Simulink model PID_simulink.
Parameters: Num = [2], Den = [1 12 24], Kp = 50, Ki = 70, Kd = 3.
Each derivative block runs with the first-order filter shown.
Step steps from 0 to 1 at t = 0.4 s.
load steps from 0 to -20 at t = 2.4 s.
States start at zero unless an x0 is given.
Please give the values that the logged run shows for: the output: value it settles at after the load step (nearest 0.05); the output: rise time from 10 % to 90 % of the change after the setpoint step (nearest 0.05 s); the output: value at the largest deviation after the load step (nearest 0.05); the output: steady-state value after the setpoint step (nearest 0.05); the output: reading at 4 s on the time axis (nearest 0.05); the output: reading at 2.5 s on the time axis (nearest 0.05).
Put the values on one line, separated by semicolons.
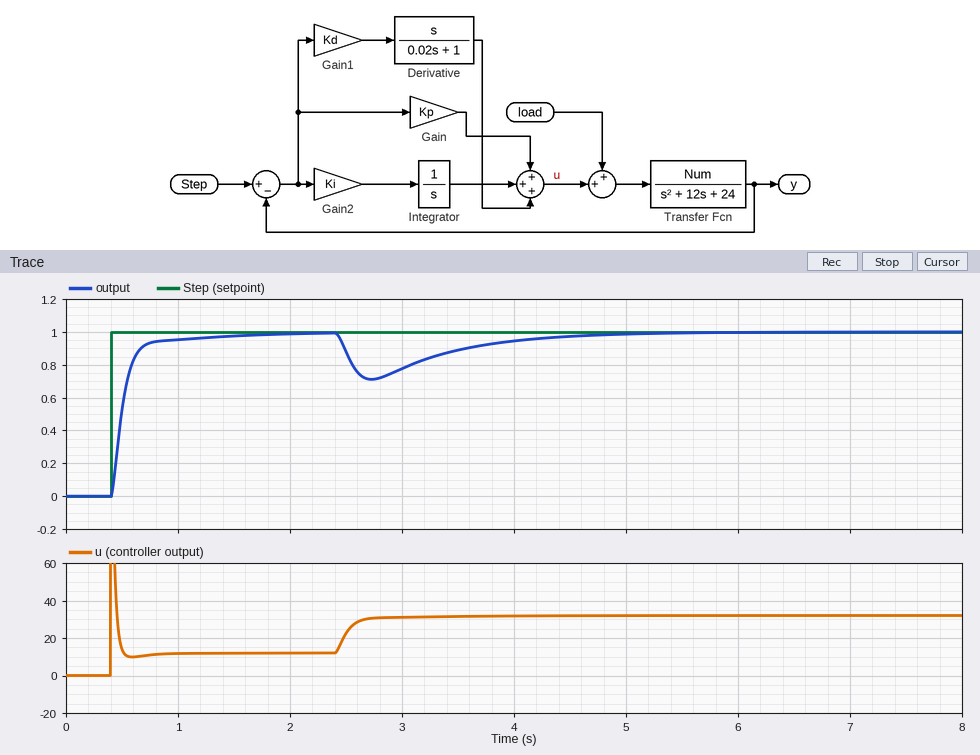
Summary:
1.00; 0.25 s; 0.70; 1.00; 0.95; 0.90
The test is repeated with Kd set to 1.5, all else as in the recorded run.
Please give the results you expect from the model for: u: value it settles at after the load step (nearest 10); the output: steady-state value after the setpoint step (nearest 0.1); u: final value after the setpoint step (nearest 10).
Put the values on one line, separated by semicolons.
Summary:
30; 1.0; 10
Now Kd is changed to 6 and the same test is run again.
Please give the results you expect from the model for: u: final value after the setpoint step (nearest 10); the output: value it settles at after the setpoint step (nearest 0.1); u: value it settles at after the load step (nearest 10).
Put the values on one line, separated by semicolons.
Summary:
10; 1.0; 30
